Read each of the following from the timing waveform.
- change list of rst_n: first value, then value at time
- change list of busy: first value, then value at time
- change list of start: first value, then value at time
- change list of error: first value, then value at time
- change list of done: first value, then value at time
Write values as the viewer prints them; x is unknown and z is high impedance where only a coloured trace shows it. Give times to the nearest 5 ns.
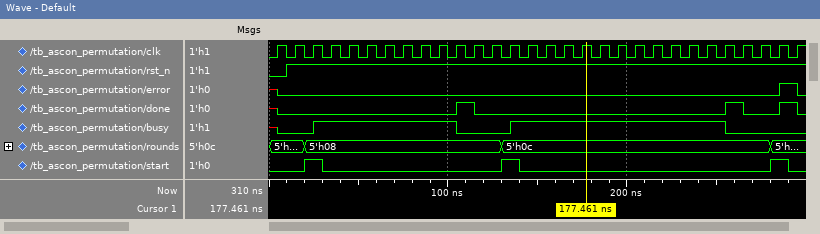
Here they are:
0, 1 at 10 ns
x, 0 at 5 ns, 1 at 25 ns, 0 at 105 ns, 1 at 135 ns, 0 at 255 ns
0, 1 at 20 ns, 0 at 30 ns, 1 at 130 ns, 0 at 140 ns, 1 at 280 ns, 0 at 290 ns
x, 0 at 5 ns, 1 at 285 ns, 0 at 295 ns
x, 0 at 5 ns, 1 at 105 ns, 0 at 115 ns, 1 at 255 ns, 0 at 265 ns, 1 at 285 ns, 0 at 295 ns
